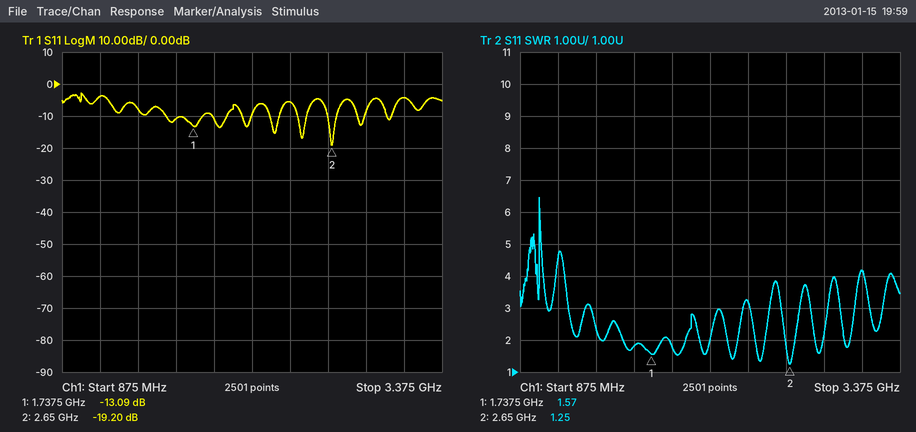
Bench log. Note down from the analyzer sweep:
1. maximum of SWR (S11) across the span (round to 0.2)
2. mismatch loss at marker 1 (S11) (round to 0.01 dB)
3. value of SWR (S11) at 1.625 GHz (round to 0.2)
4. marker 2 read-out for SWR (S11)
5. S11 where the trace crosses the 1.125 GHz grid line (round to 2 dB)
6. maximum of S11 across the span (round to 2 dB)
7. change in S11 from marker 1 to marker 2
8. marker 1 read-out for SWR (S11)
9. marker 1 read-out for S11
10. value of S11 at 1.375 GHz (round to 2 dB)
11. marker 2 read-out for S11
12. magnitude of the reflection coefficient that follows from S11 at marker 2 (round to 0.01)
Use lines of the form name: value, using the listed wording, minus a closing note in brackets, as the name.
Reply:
maximum of SWR (S11) across the span: 6.4
mismatch loss at marker 1 (S11): 0.22 dB
value of SWR (S11) at 1.625 GHz: 1.8
marker 2 read-out for SWR: 1.25
S11 where the trace crosses the 1.125 GHz grid line: -4 dB
maximum of S11 across the span: -2 dB
change in S11 from marker 1 to marker 2: -6.11 dB
marker 1 read-out for SWR: 1.57
marker 1 read-out for S11: -13.09 dB
value of S11 at 1.375 GHz: -8 dB
marker 2 read-out for S11: -19.20 dB
magnitude of the reflection coefficient that follows from S11 at marker 2: 0.11
